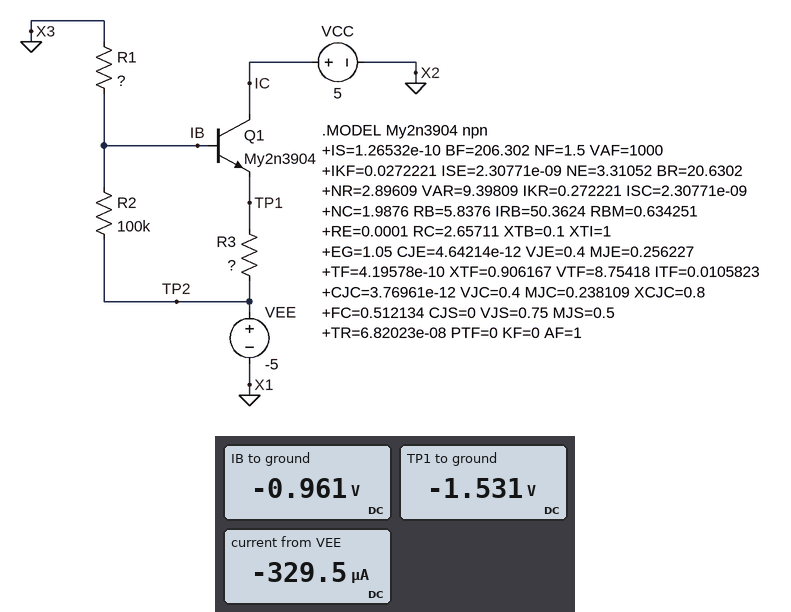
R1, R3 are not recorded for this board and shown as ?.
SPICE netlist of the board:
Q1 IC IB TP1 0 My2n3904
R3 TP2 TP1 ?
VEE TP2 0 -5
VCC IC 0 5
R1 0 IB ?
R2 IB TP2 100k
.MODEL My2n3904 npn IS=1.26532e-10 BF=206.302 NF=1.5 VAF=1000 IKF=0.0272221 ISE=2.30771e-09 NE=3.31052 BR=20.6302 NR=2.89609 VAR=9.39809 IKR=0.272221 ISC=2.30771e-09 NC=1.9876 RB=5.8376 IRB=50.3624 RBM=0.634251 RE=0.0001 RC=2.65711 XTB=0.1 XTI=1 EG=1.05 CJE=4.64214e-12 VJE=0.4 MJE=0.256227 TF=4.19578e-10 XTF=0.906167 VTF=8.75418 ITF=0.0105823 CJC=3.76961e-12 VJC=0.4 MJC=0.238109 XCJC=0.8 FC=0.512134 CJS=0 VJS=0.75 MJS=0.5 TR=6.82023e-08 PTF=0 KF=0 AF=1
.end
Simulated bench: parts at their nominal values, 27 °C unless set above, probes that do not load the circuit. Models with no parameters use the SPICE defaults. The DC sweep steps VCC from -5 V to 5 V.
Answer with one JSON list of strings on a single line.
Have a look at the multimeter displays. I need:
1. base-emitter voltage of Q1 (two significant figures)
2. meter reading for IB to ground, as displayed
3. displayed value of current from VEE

["570 mV", "-0.961 V", "-329.5 µA"]
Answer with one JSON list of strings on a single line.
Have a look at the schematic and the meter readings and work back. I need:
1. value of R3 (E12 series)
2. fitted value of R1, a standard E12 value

["12 kΩ", "22 kΩ"]
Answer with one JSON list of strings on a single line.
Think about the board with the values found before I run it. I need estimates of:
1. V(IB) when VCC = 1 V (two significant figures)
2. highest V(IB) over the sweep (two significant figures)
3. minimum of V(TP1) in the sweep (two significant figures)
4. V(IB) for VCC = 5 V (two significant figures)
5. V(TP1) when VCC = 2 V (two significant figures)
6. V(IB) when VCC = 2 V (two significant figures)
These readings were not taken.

["-960 mV", "-960 mV", "-4.9 V", "-960 mV", "-1.5 V", "-960 mV"]
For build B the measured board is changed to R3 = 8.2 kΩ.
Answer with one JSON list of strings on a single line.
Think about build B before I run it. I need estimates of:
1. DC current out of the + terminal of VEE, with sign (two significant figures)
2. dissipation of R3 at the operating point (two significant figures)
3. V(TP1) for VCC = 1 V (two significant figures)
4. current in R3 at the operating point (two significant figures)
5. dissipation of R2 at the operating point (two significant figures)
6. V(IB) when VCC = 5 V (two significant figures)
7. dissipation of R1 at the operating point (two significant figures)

["-460 µA", "1.4 mW", "-1.6 V", "420 µA", "160 µW", "-980 mV", "44 µW"]
